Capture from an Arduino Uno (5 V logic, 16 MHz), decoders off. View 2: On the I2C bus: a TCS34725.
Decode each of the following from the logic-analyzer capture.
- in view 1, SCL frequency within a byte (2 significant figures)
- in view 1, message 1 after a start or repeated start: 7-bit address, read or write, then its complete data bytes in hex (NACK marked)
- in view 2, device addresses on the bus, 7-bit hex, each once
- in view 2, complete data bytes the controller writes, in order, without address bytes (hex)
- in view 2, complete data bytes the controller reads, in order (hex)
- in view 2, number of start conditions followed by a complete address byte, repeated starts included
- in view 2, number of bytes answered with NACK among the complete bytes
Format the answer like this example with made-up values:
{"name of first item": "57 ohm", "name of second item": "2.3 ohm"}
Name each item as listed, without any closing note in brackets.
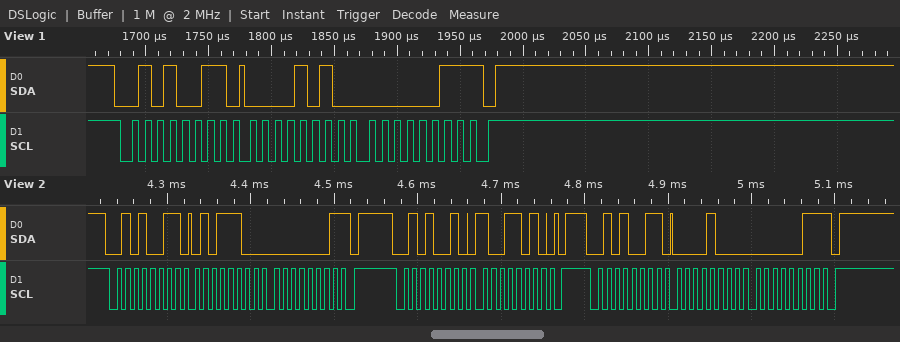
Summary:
{"in view 1, SCL frequency within a byte": "100 kHz", "in view 1, message 1 after a start or repeated start: 7-bit address, read or write, then its complete data bytes in hex": "0x29 read: 0A 03 NACK", "in view 2, device addresses on the bus, 7-bit hex, each once": "0x29", "in view 2, complete data bytes the controller writes, in order, without address bytes": "9A", "in view 2, complete data bytes the controller reads, in order": "5C 01 08 03", "in view 2, number of start conditions followed by a complete address byte, repeated starts included": "3", "in view 2, number of bytes answered with NACK among the complete bytes": "2"}
